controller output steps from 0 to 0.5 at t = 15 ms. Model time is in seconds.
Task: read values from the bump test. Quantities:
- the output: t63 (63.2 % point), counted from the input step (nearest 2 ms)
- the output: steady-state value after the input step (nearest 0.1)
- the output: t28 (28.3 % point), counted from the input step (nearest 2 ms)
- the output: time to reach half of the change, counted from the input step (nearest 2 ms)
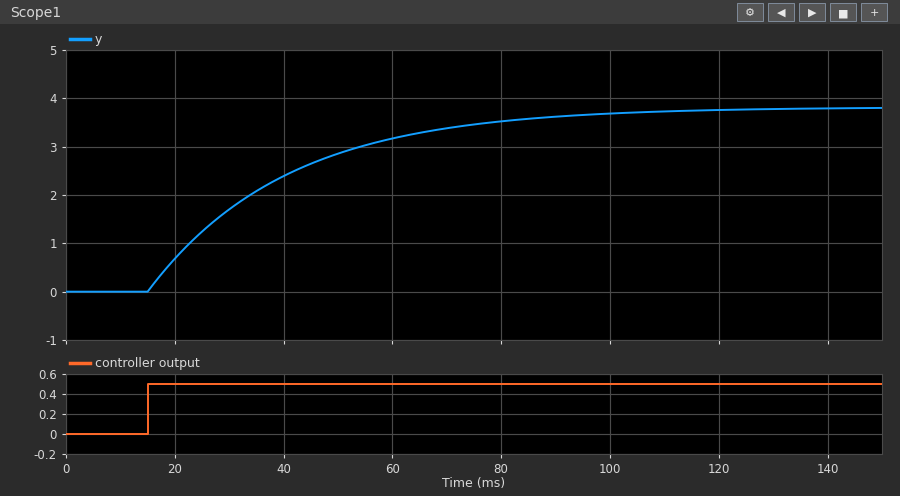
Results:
26 ms
3.8
8 ms
18 ms
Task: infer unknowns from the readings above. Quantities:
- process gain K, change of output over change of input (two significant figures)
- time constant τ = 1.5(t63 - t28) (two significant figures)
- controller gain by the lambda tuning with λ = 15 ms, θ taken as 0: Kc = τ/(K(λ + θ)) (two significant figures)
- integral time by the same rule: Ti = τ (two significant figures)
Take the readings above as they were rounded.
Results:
7.6
27 ms
0.24
27 ms
